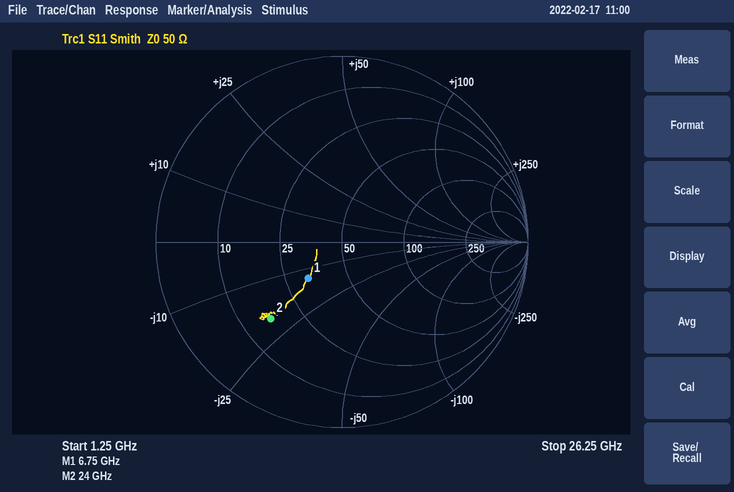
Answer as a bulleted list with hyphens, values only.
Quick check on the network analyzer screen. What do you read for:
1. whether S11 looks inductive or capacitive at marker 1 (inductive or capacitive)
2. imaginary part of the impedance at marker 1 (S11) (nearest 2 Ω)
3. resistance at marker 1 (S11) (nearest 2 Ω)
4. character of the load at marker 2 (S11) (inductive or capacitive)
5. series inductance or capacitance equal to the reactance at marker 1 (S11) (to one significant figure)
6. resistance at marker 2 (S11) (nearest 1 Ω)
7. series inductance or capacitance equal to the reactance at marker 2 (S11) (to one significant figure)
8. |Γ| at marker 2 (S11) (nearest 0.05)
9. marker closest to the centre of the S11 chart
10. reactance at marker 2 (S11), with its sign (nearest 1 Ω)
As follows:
- capacitive
- -14 Ω
- 32 Ω
- capacitive
- 2 pF
- 16 Ω
- 300 fF
- 0.55
- marker 1
- -20 Ω
